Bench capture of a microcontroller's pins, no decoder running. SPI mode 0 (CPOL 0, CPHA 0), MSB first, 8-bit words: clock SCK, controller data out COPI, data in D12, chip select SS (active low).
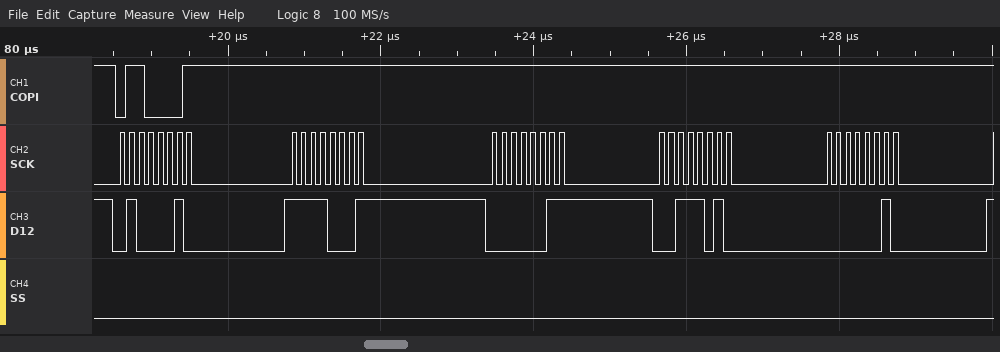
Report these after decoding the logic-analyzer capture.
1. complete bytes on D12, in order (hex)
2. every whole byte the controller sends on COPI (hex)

0x42 0xF1 0x03 0x3A 0x02
0x61 0xFF 0xFF 0xFF 0xFF
